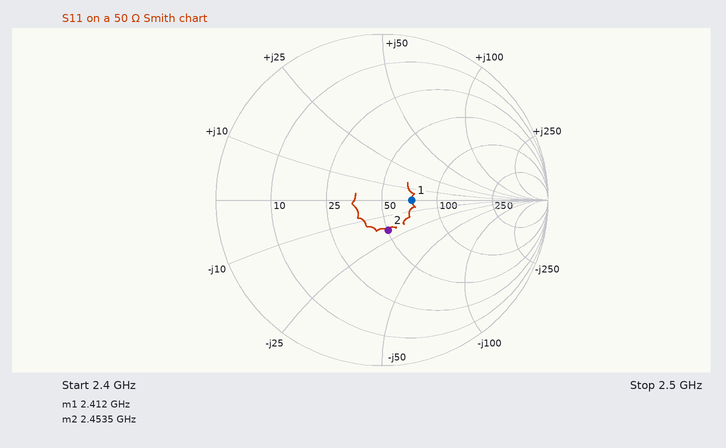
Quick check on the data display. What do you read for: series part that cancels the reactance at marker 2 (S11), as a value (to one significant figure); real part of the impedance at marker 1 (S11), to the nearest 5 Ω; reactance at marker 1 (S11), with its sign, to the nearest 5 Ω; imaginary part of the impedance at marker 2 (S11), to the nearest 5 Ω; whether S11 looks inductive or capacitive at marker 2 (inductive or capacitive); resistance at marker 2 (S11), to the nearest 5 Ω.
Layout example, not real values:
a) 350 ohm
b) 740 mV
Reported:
a) 1 nH
b) 70 Ω
c) 0 Ω
d) -20 Ω
e) capacitive
f) 50 Ω
